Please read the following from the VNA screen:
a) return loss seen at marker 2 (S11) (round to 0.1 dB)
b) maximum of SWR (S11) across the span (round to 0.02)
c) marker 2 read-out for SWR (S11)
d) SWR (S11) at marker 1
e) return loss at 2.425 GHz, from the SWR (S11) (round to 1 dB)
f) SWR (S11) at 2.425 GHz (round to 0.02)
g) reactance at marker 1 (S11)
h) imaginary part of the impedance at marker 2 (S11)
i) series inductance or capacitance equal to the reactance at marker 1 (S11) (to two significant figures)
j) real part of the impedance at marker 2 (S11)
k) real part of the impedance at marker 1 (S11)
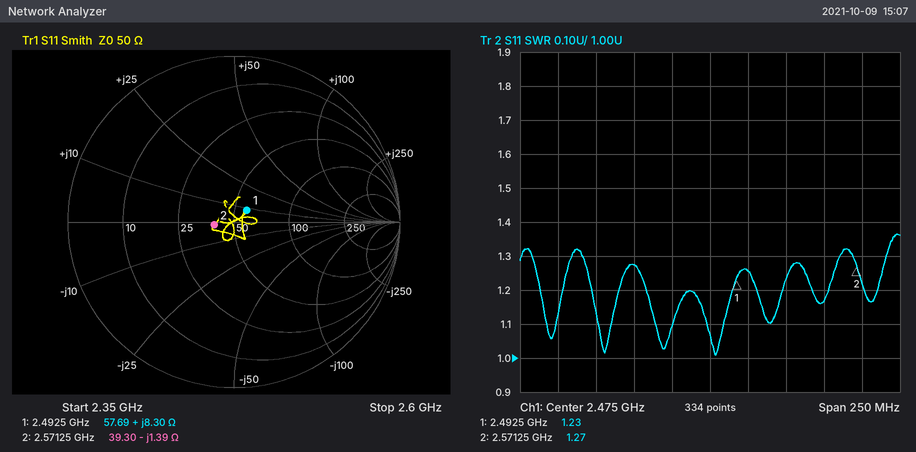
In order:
18.4 dB
1.36
1.27
1.23
18 dB
1.28
+8.30 Ω
-1.39 Ω
530 pH
39.30 Ω
57.69 Ω
